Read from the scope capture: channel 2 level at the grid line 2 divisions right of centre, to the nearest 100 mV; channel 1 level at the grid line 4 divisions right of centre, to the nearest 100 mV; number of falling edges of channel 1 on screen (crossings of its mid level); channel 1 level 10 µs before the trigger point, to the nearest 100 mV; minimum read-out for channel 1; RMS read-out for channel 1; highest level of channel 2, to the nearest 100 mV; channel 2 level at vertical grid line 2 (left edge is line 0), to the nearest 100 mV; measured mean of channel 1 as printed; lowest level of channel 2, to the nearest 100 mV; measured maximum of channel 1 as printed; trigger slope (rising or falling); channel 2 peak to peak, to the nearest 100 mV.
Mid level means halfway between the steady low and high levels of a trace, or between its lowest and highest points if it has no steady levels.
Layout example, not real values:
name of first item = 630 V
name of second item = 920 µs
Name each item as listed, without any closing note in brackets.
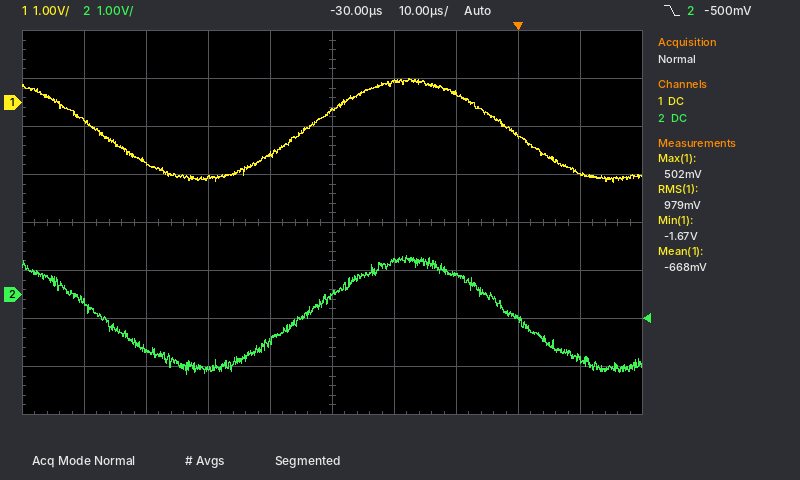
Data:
channel 2 level at the grid line 2 divisions right of centre, to the nearest 100 mV = 400 mV
channel 1 level at the grid line 4 divisions right of centre, to the nearest 100 mV = -1.5 V
number of falling edges of channel 1 on screen = 2
channel 1 level 10 µs before the trigger point, to the nearest 100 mV = 200 mV
minimum read-out for channel 1 = -1.67 V
RMS read-out for channel 1 = 979 mV
highest level of channel 2, to the nearest 100 mV = 800 mV
channel 2 level at vertical grid line 2 (left edge is line 0), to the nearest 100 mV = -1.1 V
measured mean of channel 1 as printed = -668 mV
lowest level of channel 2, to the nearest 100 mV = -1.7 V
measured maximum of channel 1 as printed = 502 mV
trigger slope = falling
channel 2 peak to peak, to the nearest 100 mV = 2.5 V
